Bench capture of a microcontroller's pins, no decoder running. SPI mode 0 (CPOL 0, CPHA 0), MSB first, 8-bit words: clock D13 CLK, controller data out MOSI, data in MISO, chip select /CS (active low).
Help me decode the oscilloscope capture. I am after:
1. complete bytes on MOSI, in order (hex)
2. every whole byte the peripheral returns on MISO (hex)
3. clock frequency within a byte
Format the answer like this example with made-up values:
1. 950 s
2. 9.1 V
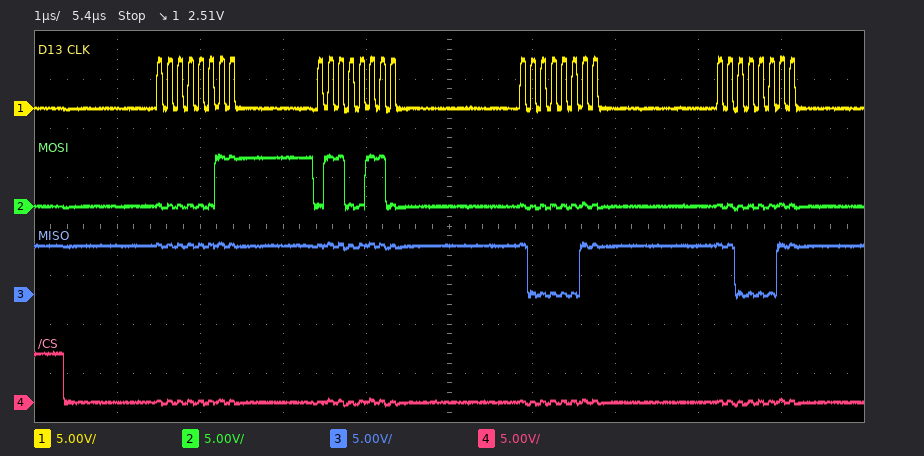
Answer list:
1. 03 66 00 00
2. FF FF 83 C3
3. 8 MHz
